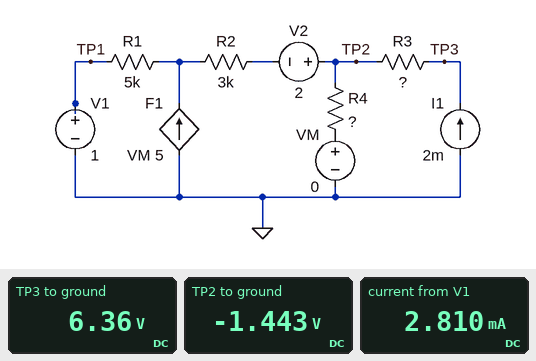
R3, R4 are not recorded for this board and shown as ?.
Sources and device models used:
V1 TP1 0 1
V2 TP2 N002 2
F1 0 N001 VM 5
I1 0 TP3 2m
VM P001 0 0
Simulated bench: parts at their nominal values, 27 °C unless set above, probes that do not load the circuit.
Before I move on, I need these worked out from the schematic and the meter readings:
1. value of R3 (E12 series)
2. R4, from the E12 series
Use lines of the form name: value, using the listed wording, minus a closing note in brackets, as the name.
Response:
value of R3: 3.9 kΩ
R4, from the E12 series: 1.2 kΩ
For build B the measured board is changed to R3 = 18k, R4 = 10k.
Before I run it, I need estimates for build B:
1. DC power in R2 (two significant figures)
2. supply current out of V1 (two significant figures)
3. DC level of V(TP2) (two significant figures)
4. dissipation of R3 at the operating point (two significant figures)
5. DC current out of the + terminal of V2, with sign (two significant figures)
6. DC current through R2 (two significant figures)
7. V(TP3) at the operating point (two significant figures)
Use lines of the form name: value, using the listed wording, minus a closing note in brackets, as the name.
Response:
DC power in R2: 67 mW
supply current out of V1: 8.9 mA
DC level of V(TP2): -27 V
dissipation of R3 at the operating point: 72 mW
DC current out of the + terminal of V2, with sign: -4.7 mA
DC current through R2: 4.7 mA
V(TP3) at the operating point: 8.9 V
